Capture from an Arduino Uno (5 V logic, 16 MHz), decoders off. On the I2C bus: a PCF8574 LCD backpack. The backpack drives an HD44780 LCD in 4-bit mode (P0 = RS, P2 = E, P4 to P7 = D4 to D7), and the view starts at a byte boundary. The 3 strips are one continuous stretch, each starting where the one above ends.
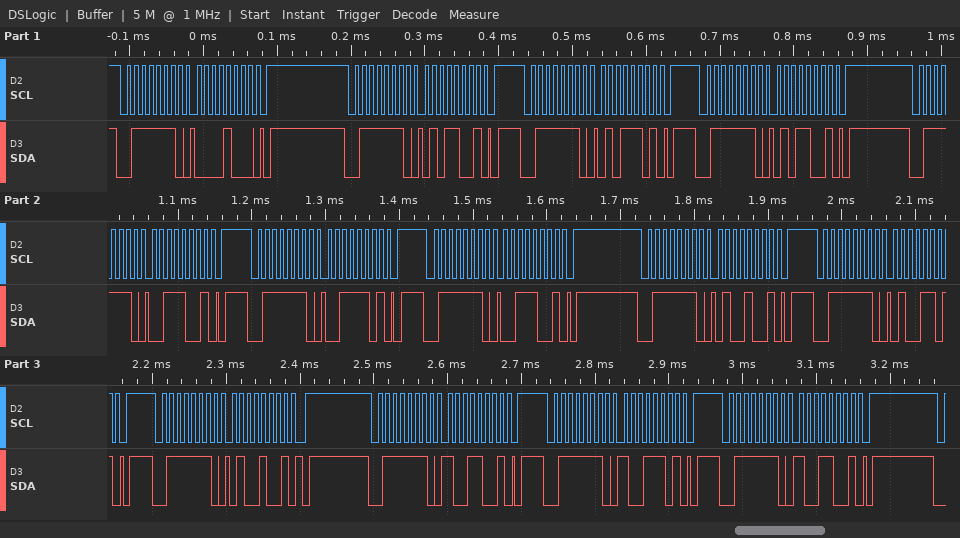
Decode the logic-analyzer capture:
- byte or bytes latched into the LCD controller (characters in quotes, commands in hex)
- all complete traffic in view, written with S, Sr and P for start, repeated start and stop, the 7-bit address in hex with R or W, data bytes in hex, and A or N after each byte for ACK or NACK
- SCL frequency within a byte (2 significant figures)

'S' 'I'
S 3FW A 08 A P S 3FW A 59 A P S 3FW A 5D A P S 3FW A 59 A P S 3FW A 39 A P S 3FW A 3D A P S 3FW A 39 A P S 3FW A 49 A P S 3FW A 4D A P S 3FW A 49 A P S 3FW A 99 A P S 3FW A 9D A P S 3FW A 99 A P
100 kHz
